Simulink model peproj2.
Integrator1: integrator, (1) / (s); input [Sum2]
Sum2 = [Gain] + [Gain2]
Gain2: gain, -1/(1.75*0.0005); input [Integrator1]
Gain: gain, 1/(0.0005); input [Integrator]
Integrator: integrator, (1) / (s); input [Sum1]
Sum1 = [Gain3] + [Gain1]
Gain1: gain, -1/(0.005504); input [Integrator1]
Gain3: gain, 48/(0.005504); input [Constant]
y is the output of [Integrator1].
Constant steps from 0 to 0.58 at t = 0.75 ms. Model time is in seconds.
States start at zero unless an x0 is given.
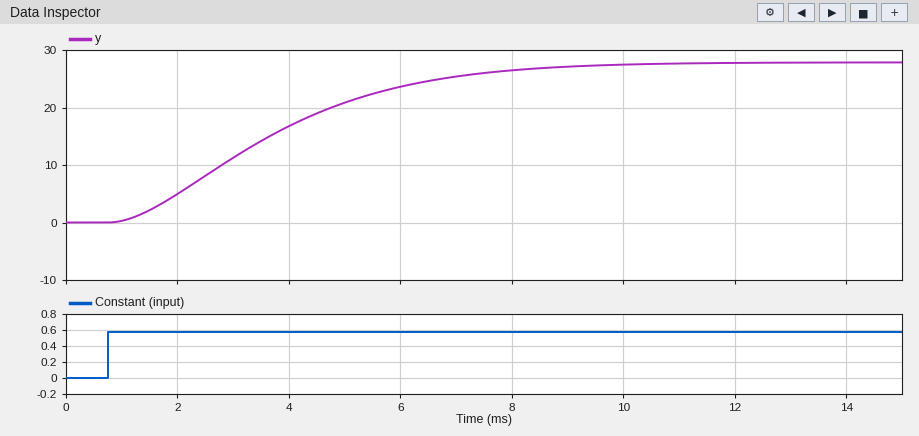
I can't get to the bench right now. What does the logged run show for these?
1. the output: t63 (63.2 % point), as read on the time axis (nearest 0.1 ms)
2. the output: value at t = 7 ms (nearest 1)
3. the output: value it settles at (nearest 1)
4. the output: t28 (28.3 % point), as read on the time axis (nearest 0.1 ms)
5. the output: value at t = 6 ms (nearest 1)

4.2 ms
25
28
2.5 ms
24
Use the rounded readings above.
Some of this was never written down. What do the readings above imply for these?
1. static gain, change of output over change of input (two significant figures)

48
